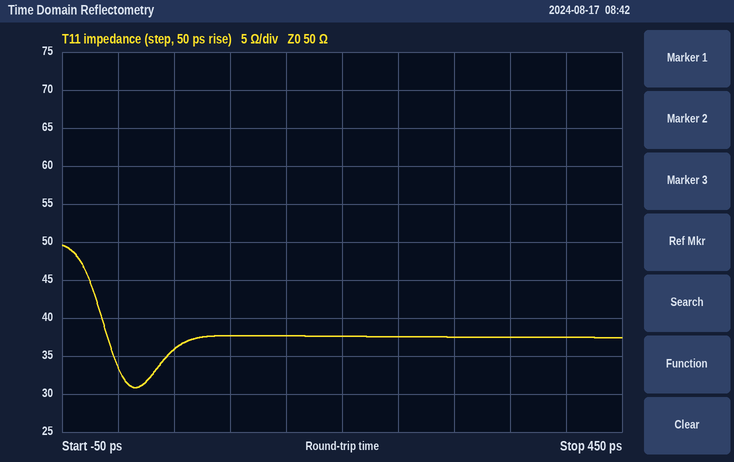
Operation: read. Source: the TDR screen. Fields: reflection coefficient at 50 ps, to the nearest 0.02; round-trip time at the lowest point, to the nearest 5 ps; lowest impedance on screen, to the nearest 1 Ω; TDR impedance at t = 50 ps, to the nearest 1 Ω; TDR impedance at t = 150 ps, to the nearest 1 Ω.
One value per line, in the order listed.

-0.16
15 ps
31 Ω
36 Ω
38 Ω
